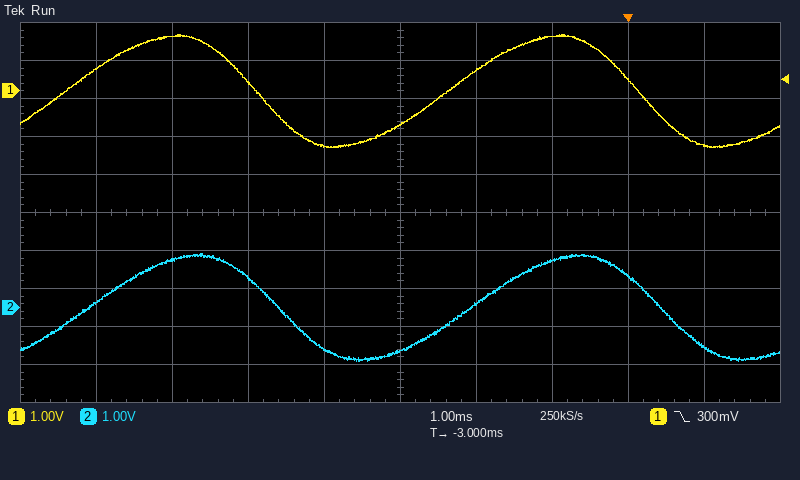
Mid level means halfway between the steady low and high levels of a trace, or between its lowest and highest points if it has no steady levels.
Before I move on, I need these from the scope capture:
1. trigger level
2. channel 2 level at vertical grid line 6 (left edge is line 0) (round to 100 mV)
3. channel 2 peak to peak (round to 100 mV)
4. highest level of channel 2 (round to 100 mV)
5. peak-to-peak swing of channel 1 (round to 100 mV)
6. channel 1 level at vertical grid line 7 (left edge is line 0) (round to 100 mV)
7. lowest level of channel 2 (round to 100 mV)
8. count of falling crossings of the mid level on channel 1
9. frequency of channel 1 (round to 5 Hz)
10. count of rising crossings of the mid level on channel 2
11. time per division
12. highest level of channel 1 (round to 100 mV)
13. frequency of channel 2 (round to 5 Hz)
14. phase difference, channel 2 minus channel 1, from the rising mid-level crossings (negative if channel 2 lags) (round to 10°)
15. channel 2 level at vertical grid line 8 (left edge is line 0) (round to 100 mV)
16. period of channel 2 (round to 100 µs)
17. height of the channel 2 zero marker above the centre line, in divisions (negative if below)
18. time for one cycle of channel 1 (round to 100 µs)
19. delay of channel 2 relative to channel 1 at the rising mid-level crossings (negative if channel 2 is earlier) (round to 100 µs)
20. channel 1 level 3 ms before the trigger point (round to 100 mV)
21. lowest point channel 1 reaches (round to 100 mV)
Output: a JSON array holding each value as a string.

["300 mV", "100 mV", "2.8 V", "1.4 V", "3.0 V", "1.4 V", "-1.4 V", "2", "200 Hz", "2", "1 ms", "1.5 V", "200 Hz", "-20°", "800 mV", "5.0 ms", "-2.5 div", "5.0 ms", "+300 µs", "-900 mV", "-1.5 V"]
